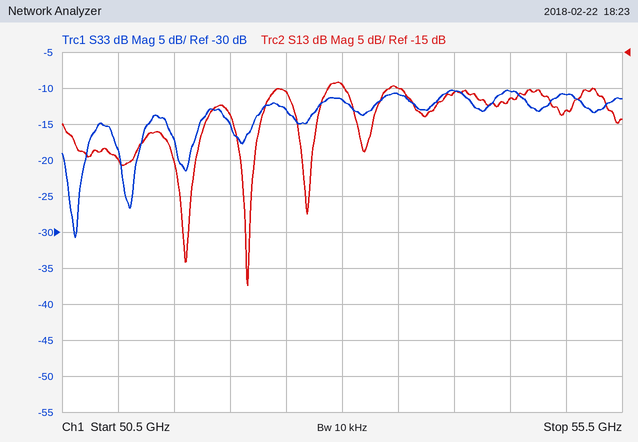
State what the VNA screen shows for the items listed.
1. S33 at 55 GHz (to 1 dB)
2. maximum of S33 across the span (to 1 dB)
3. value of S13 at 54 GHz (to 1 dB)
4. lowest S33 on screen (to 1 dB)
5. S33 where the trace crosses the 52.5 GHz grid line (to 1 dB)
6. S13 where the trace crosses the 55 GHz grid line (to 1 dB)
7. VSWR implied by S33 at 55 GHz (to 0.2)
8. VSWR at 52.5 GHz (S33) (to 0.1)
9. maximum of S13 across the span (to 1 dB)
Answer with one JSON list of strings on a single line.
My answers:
["-11 dB", "-10 dB", "-21 dB", "-31 dB", "-13 dB", "-23 dB", "1.8", "1.6", "-19 dB"]
